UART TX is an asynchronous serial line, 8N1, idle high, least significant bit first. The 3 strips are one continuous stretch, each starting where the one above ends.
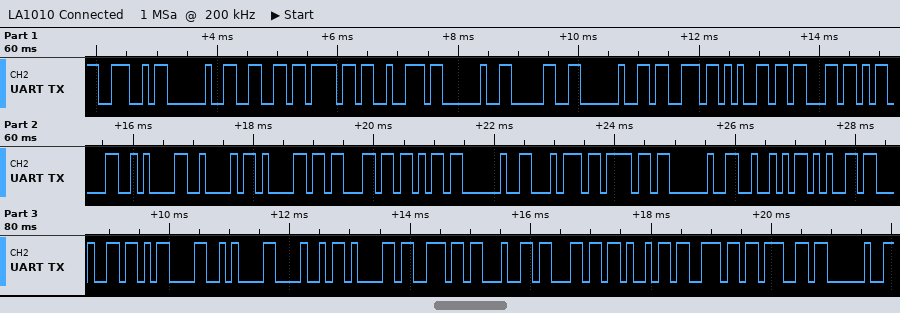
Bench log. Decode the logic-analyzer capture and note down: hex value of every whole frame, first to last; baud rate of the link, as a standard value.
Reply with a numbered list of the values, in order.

1. 4E 20 66 6F 72 20 30 20 73 65 63 0D 0A 42 61 63 6B 20 74 6F 20 52 65 64 0D 0A 48 61 6E 64 6C 69 6E 67 20
2. 9600 baud
